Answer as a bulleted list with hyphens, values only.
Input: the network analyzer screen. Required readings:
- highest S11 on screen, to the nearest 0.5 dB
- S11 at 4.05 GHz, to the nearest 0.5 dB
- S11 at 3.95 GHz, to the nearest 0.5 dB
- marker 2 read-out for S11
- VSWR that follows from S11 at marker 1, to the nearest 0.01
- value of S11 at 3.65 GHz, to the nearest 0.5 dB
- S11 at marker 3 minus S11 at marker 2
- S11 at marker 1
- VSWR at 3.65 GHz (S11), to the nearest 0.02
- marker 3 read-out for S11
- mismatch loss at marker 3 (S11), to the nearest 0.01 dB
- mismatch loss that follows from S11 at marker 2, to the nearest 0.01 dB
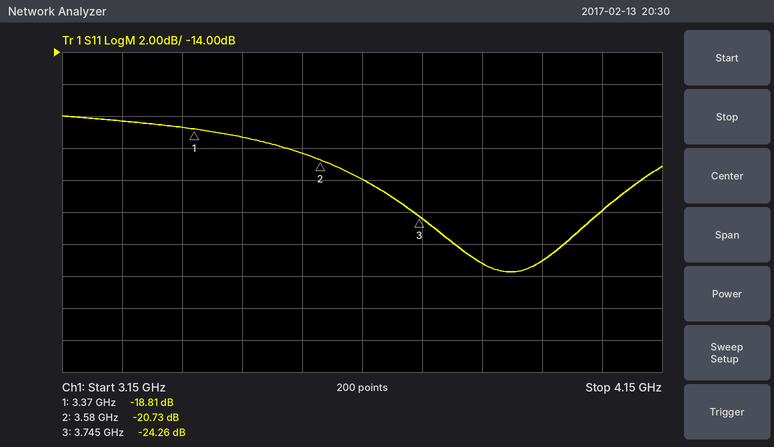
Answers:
- -18.0 dB
- -24.0 dB
- -27.0 dB
- -20.73 dB
- 1.26
- -22.0 dB
- -3.53 dB
- -18.81 dB
- 1.18
- -24.26 dB
- 0.02 dB
- 0.04 dB
